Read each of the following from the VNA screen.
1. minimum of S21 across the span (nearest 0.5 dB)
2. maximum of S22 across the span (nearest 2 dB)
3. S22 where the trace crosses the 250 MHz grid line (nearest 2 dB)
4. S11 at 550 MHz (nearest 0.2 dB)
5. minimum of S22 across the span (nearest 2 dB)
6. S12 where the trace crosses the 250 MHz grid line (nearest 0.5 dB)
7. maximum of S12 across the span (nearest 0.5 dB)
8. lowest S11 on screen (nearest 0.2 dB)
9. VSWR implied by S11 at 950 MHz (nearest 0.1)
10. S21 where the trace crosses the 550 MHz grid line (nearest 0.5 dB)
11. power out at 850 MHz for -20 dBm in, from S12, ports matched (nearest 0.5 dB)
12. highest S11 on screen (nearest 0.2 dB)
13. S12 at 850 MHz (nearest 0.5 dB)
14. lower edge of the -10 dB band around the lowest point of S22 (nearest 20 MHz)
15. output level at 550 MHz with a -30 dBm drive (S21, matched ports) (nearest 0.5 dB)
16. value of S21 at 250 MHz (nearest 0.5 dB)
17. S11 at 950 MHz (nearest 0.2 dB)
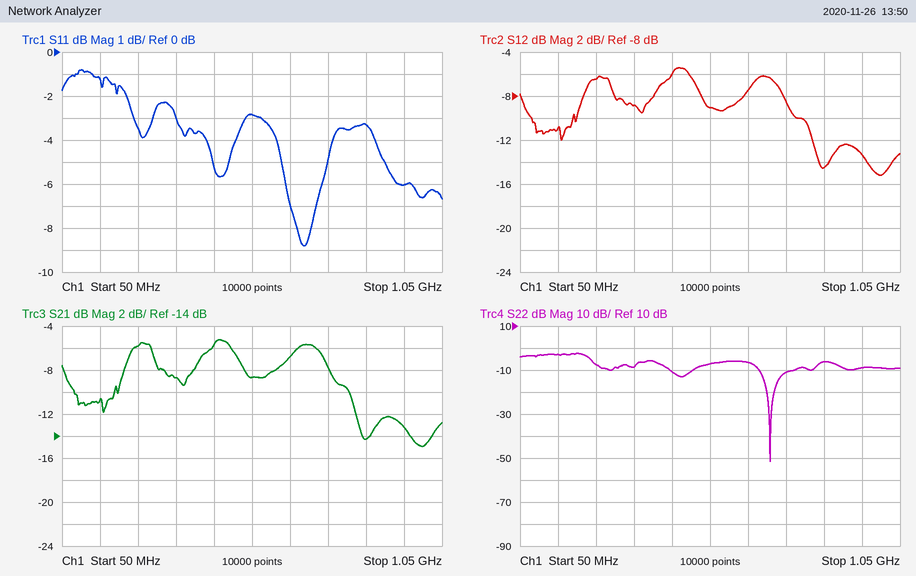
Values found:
-15.0 dB
-2 dB
-8 dB
-2.8 dB
-52 dB
-6.5 dB
-5.5 dB
-8.8 dB
3.0
-8.5 dB
-34.5 dBm
-0.8 dB
-14.5 dB
680 MHz
-38.5 dBm
-6.0 dB
-6.0 dB
